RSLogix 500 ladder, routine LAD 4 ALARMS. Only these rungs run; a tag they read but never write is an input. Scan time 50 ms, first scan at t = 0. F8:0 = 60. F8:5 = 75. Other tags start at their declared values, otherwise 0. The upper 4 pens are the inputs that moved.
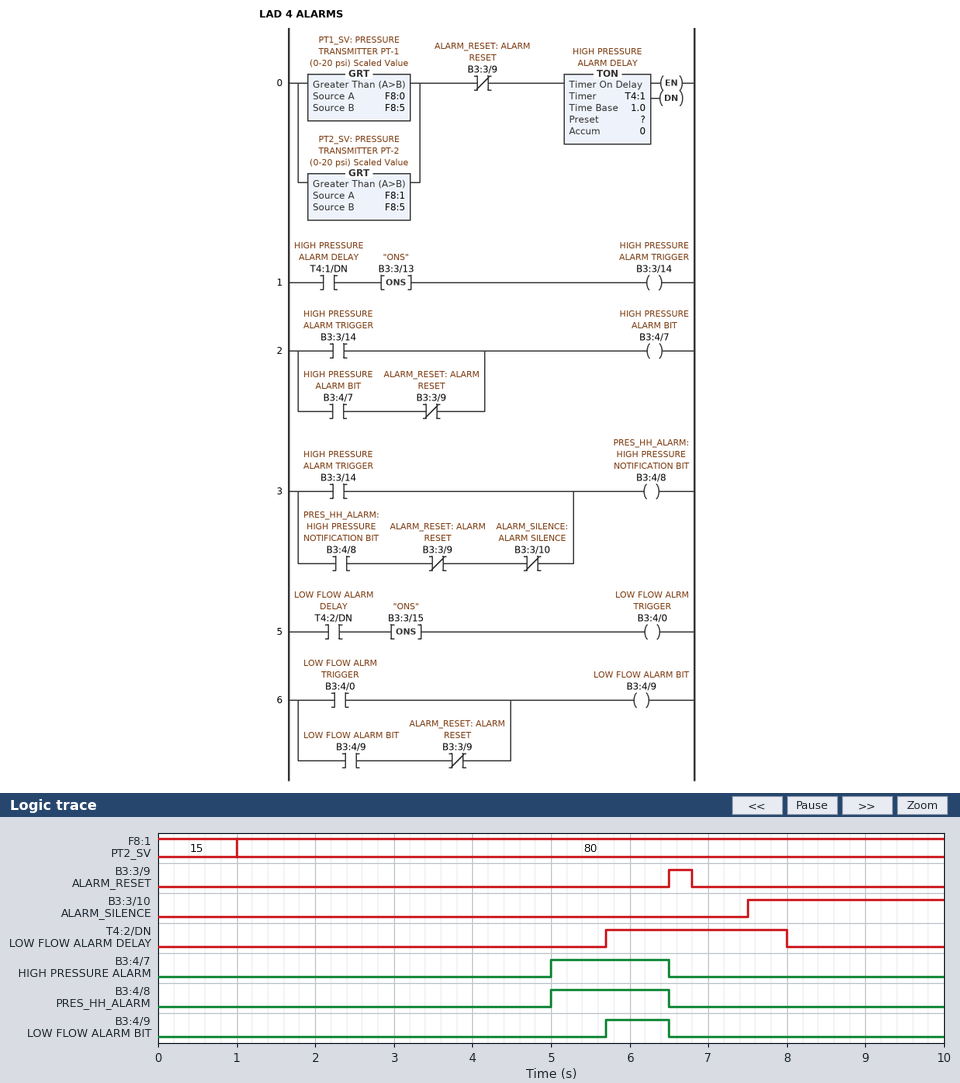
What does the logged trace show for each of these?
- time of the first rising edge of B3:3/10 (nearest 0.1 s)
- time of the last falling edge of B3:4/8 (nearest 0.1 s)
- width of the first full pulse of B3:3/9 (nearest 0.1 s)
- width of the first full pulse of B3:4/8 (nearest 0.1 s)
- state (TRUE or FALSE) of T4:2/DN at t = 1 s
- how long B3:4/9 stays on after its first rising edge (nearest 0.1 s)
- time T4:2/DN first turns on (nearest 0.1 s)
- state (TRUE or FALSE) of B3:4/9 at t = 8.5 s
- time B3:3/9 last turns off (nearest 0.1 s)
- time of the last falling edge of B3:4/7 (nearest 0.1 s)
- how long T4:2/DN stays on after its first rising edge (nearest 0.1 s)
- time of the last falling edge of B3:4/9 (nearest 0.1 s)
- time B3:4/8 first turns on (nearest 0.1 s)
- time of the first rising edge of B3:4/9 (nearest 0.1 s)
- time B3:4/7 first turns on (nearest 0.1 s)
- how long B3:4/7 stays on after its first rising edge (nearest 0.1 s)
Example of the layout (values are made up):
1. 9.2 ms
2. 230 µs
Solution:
1. 7.5 s
2. 6.5 s
3. 0.3 s
4. 1.5 s
5. FALSE
6. 0.8 s
7. 5.7 s
8. FALSE
9. 6.8 s
10. 6.5 s
11. 2.3 s
12. 6.5 s
13. 5.0 s
14. 5.7 s
15. 5.0 s
16. 1.5 s
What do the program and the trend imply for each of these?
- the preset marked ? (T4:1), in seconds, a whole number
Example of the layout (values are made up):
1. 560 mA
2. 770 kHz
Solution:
1. 4 s
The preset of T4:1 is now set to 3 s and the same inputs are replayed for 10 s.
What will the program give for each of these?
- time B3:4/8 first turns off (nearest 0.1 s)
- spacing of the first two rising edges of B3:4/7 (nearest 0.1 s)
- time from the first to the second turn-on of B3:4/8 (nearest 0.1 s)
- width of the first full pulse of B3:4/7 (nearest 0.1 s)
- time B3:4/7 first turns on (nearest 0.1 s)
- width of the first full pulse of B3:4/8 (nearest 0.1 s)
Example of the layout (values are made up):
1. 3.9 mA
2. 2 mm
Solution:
1. 6.5 s
2. 5.8 s
3. 5.8 s
4. 2.5 s
5. 4.0 s
6. 2.5 s
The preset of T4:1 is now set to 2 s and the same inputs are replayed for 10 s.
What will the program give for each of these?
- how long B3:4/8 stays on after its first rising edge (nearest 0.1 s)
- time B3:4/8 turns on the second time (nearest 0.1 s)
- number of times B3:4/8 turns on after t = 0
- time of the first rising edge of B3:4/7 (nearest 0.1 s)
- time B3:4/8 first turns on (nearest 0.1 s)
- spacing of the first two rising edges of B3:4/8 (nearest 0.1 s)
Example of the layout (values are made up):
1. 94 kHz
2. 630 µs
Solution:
1. 3.5 s
2. 8.8 s
3. 2
4. 3.0 s
5. 3.0 s
6. 5.8 s
